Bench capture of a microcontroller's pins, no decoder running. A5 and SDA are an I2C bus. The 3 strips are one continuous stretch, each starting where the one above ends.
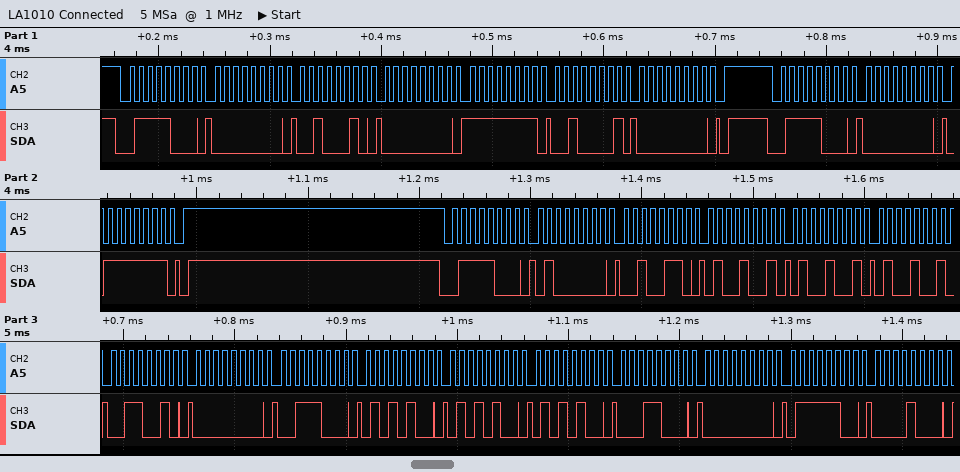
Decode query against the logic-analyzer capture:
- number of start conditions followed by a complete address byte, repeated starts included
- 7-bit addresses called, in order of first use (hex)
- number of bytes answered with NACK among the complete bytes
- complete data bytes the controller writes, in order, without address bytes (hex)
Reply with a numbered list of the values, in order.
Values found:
1. 3
2. 0x3C
3. 0
4. 00 22 00 FF 21 00 00 7F 40 26 49 49 49 32 00 38 54 54 54 18 00 7C 08
